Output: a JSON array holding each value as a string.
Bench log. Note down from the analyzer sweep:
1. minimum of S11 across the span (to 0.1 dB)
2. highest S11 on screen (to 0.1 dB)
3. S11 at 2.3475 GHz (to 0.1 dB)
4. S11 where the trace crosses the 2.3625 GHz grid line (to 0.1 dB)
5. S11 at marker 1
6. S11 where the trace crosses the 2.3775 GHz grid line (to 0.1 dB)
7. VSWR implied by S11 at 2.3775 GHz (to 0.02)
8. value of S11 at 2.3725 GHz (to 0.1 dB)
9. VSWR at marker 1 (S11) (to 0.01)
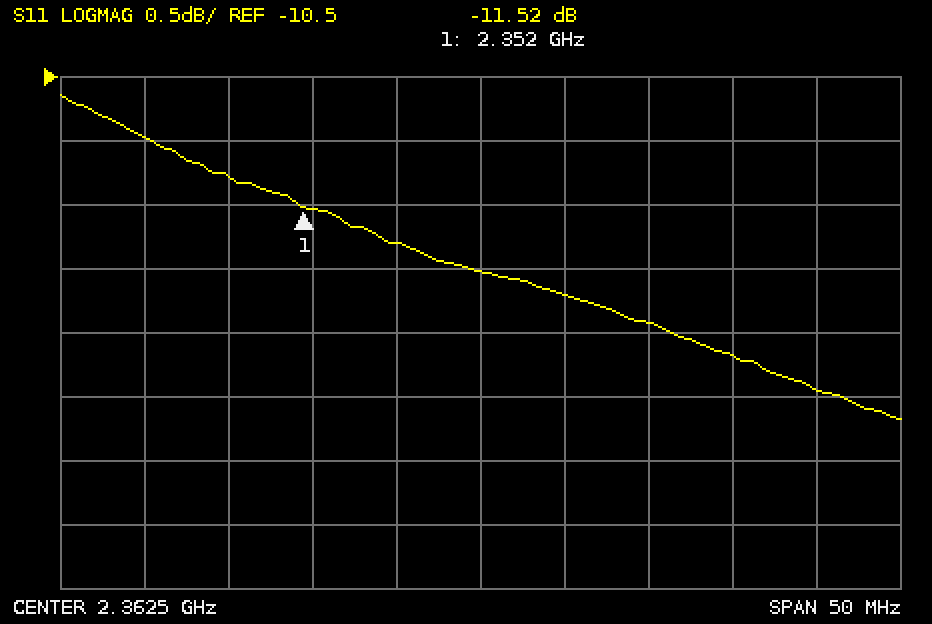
["-13.2 dB", "-10.6 dB", "-11.3 dB", "-12.0 dB", "-11.52 dB", "-12.7 dB", "1.60", "-12.4 dB", "1.72"]
